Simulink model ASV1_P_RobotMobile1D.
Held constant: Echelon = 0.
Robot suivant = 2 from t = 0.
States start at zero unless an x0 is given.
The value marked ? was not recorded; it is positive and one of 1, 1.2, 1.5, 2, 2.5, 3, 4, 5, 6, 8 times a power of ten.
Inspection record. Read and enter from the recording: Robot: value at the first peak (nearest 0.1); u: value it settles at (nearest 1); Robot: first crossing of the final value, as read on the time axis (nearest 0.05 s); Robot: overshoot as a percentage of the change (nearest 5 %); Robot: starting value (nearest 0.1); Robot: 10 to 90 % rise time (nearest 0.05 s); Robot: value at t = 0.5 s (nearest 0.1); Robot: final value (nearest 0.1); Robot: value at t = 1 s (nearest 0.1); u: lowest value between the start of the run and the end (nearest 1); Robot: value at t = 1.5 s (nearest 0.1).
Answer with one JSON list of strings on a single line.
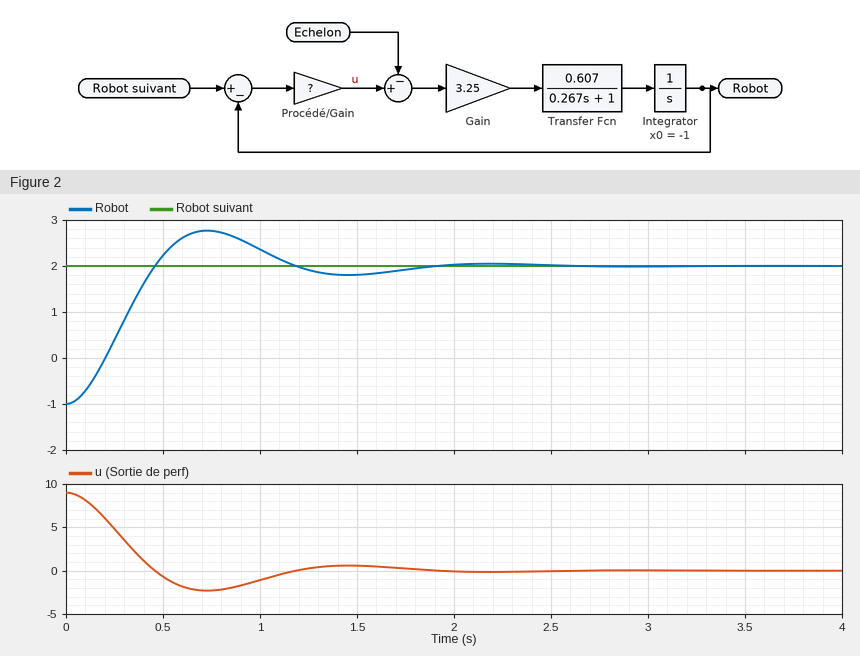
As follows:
["2.8", "0", "0.45 s", "25 %", "-1.0", "0.30 s", "2.2", "2.0", "2.4", "-2", "1.8"]
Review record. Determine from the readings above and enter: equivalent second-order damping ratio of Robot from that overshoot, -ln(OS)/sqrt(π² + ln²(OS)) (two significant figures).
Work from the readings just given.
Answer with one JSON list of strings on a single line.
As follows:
["0.40"]
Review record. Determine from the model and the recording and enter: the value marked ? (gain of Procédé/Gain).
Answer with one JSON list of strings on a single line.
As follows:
["3"]
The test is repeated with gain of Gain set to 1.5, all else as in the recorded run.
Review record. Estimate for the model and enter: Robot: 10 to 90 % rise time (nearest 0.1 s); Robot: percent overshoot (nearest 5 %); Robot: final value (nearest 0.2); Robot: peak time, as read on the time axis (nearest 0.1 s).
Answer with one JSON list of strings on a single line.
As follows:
["0.6 s", "10 %", "2.0", "1.2 s"]
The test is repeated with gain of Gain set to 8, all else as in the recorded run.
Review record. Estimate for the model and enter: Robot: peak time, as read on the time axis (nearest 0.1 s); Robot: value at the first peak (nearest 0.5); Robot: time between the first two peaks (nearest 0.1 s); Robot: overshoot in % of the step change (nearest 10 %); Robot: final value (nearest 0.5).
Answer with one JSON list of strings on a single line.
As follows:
["0.4 s", "3.5", "0.9 s", "40 %", "2.0"]
